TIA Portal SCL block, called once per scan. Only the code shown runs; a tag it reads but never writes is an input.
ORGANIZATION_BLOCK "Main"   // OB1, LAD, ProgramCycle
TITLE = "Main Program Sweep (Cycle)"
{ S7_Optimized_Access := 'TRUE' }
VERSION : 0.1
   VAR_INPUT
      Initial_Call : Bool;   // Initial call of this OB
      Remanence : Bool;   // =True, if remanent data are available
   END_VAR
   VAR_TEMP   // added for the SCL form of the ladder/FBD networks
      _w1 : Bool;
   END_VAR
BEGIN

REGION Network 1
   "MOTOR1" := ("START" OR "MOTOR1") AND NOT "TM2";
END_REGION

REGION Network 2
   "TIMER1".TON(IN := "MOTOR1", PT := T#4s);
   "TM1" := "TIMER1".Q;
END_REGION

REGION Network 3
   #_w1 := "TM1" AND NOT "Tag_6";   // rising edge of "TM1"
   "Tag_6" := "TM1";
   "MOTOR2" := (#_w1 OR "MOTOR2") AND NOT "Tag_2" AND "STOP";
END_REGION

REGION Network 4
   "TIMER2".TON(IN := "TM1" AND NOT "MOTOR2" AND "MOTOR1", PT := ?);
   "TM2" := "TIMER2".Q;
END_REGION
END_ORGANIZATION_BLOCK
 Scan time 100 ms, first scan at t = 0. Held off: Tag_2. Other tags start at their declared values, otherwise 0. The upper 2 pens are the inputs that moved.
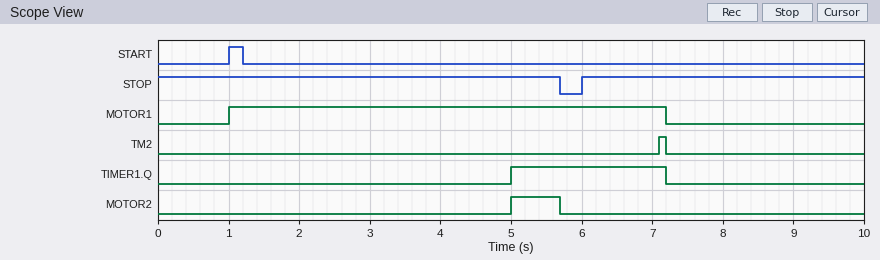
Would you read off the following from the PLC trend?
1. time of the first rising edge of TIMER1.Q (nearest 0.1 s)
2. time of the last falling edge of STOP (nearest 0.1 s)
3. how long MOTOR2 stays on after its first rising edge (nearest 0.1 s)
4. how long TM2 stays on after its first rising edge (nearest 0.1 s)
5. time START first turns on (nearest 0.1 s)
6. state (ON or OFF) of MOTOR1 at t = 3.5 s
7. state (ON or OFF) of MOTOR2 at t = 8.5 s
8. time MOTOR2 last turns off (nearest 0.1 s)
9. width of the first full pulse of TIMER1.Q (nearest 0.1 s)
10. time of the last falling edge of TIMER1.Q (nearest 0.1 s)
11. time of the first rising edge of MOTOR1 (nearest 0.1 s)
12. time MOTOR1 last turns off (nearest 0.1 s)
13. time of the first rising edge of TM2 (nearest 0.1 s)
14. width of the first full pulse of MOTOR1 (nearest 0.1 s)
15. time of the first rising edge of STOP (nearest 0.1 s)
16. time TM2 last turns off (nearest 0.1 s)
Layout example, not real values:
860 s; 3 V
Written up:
5.0 s; 5.7 s; 0.7 s; 0.1 s; 1.0 s; ON; OFF; 5.7 s; 2.2 s; 7.2 s; 1.0 s; 7.2 s; 7.1 s; 6.2 s; 6.0 s; 7.2 s
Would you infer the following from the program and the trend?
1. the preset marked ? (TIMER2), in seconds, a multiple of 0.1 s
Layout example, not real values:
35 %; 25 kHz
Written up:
1.4 s
